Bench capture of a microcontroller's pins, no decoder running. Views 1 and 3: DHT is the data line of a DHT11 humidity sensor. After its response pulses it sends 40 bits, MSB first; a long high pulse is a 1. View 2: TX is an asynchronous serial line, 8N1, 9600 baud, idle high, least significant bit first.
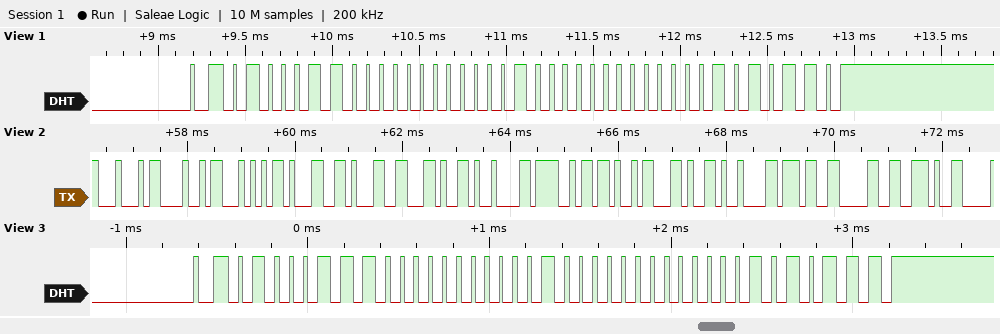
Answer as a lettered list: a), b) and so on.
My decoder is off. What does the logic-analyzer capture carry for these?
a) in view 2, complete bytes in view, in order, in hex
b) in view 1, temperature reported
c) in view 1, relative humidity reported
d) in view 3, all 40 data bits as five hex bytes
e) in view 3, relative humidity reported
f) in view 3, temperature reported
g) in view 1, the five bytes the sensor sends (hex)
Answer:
a) 44 48 54 31 31 2C 09 4F 4B 2C 09 37 30 2E
b) 16.0 °C
c) 70 %
d) 47 00 10 00 57
e) 71 %
f) 16.0 °C
g) 46 00 10 00 56
